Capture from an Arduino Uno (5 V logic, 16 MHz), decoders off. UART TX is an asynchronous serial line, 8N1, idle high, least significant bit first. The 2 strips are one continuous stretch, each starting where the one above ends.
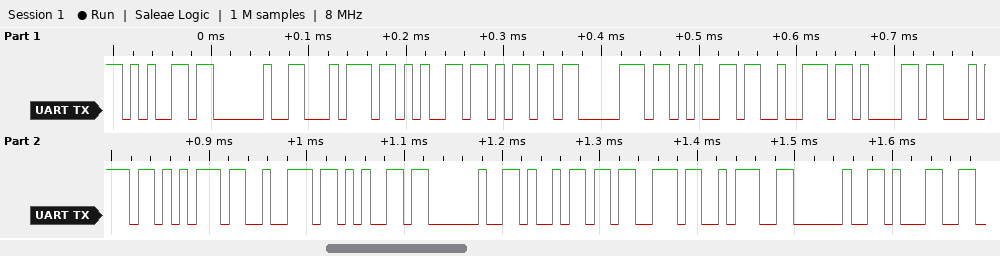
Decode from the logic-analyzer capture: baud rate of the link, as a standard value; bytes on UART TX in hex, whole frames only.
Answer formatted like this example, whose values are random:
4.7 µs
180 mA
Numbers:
115200 baud
65 20 74 65 6D 70 65 72 61 74 75 72 65 20 69 73 3A 20 31
